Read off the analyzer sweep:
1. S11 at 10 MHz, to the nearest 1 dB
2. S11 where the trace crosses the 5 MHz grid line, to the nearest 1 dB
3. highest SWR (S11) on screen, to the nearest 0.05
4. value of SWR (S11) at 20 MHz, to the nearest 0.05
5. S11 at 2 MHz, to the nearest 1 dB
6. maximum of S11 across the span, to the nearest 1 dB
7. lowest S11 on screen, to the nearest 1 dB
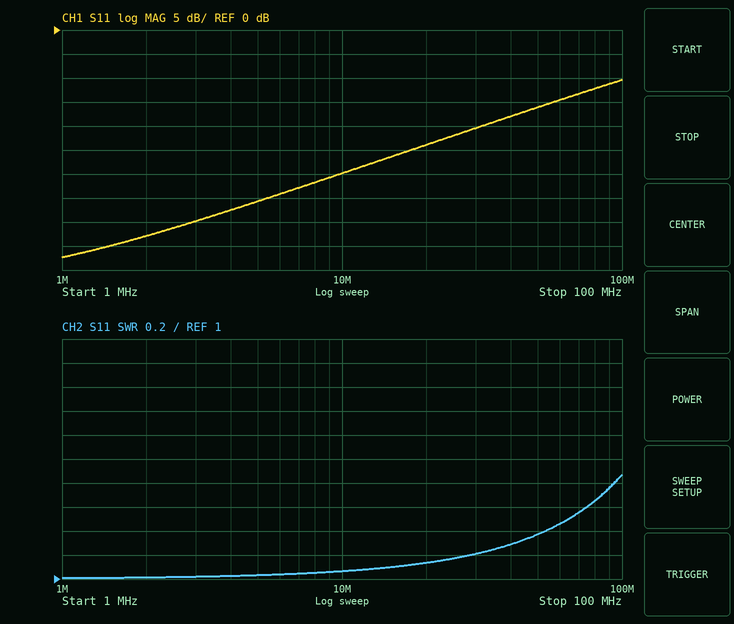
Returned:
-30 dB
-36 dB
1.85
1.15
-43 dB
-10 dB
-47 dB
